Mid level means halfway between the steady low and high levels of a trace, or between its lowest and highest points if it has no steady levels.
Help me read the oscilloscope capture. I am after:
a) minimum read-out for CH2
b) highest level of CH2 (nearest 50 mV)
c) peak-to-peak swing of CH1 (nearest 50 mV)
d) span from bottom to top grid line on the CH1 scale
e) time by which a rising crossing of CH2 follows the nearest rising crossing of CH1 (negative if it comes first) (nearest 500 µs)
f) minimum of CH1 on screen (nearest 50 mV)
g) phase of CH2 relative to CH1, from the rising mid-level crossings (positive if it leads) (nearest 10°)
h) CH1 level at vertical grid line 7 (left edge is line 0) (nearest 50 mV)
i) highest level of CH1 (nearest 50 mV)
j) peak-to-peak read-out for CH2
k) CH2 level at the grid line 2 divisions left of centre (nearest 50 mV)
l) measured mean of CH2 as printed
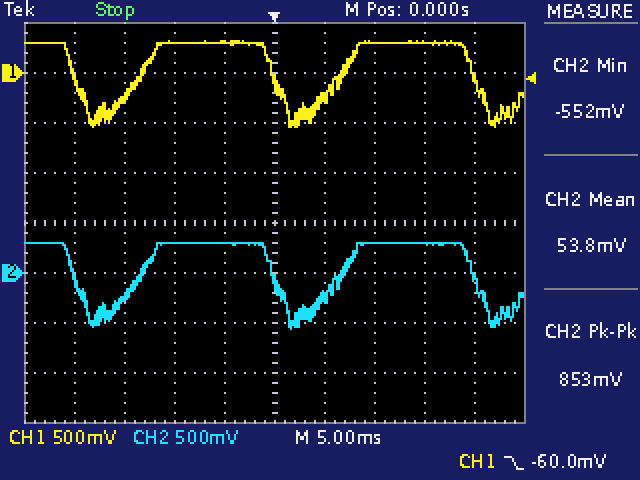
-552 mV
300 mV
850 mV
4 V
0.0 ms
-550 mV
0°
300 mV
300 mV
853 mV
300 mV
53.8 mV
